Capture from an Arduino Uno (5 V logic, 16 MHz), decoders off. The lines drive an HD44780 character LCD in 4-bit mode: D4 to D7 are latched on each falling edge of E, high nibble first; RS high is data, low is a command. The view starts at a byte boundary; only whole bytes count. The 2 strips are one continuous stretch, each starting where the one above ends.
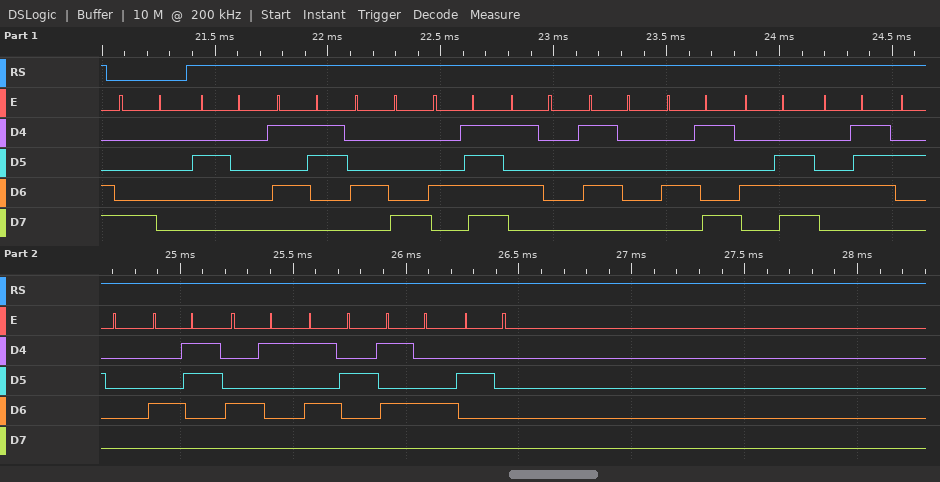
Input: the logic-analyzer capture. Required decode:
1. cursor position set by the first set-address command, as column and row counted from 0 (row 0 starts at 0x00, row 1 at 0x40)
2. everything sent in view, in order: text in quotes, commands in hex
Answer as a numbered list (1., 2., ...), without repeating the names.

1. column 0, row 0
2. 0x80 " SHOPPING CART "
